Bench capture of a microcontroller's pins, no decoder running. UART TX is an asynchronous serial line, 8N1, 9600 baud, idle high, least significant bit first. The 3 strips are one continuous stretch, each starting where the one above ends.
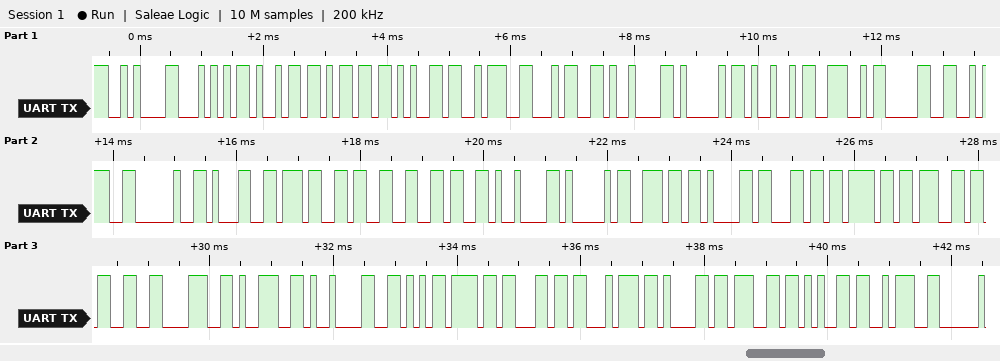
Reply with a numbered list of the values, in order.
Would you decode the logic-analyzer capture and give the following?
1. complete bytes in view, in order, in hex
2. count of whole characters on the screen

1. 0A 54 69 6D 65 3A 34 09 41 49 4E 30 3A 20 31 37 33 36 09 41 6E 61 6C 6F 67 33 38 39 09 56 6F 6C 74 61 67 65 3A
2. 37
